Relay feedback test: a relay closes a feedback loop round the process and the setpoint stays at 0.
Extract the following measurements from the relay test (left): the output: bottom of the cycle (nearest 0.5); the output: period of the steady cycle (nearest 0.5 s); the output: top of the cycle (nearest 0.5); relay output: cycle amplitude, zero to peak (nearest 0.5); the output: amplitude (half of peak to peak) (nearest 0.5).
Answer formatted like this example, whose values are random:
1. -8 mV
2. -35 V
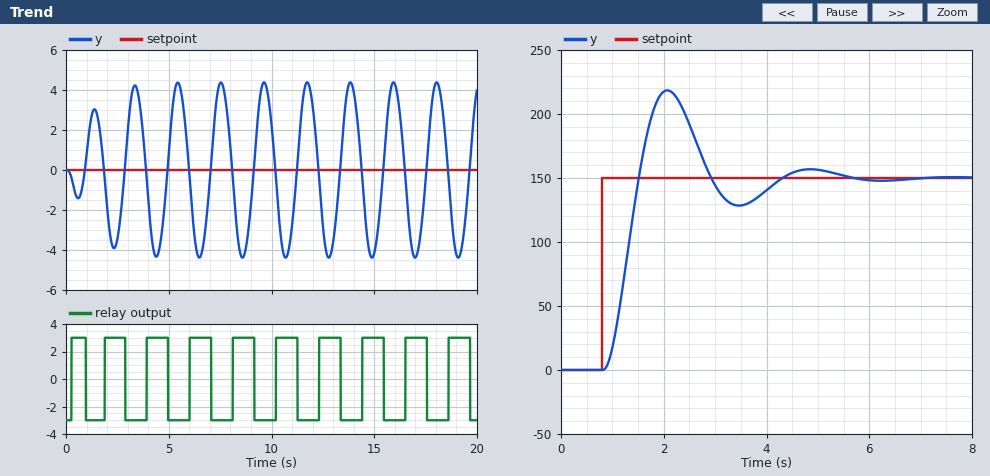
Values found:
1. -4.5
2. 2.0 s
3. 4.5
4. 3.0
5. 4.5
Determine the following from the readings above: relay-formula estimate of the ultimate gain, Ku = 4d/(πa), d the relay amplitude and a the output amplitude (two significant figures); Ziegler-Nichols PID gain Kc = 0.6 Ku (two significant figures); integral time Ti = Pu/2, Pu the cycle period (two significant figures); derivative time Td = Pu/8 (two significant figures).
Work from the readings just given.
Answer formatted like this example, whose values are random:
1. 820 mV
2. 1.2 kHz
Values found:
1. 0.85
2. 0.51
3. 1.0 s
4. 0.25 s
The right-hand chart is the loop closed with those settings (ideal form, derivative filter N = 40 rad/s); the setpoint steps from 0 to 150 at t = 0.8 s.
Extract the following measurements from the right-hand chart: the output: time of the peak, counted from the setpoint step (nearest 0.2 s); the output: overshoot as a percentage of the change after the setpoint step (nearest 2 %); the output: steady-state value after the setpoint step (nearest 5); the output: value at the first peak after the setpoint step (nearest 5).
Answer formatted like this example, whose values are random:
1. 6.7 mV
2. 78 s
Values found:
1. 1.2 s
2. 46 %
3. 150
4. 220
